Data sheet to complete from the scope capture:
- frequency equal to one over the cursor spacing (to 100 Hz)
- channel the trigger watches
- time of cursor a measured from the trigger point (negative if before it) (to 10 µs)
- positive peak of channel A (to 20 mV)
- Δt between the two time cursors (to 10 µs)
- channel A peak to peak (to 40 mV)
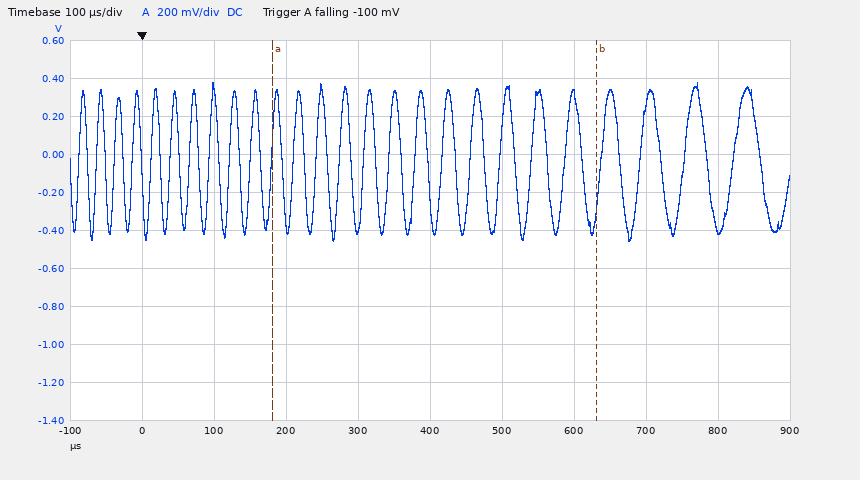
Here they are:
2.2 kHz
channel A
+180 µs
380 mV
450 µs
840 mV
